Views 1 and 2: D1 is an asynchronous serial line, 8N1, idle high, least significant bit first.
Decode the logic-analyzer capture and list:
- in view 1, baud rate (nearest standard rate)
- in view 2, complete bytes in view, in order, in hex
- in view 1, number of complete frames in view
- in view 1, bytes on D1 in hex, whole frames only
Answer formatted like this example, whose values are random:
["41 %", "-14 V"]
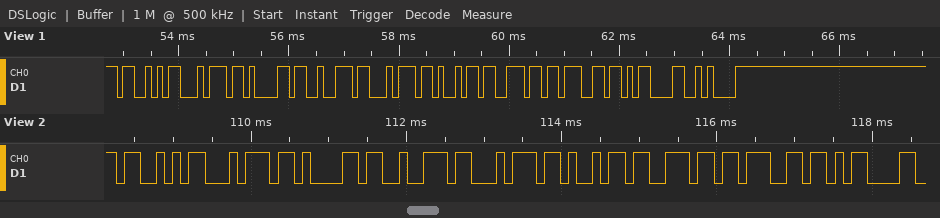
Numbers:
["9600 baud", "53 74 61 72 74 69 6E 67 0D", "10", "0x53 0x74 0x61 0x72 0x74 0x69 0x6E 0x67 0x0D 0x0A"]
